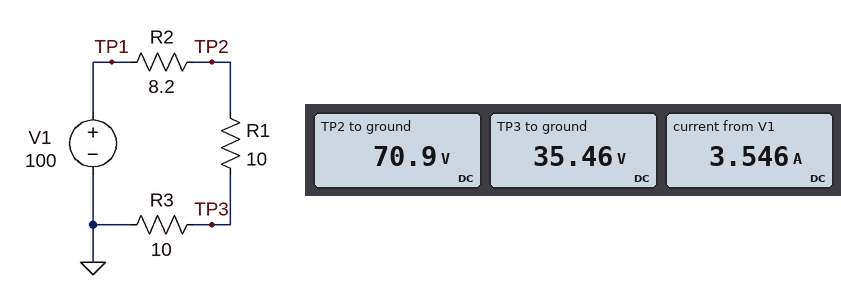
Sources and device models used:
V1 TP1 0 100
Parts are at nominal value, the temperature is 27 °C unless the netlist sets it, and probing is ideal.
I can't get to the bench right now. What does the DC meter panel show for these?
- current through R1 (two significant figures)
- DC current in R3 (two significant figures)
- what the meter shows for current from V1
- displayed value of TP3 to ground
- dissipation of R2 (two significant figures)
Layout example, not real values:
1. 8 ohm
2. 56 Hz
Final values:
1. 3.5 A
2. 3.5 A
3. 3.546 A
4. 35.46 V
5. 100 W
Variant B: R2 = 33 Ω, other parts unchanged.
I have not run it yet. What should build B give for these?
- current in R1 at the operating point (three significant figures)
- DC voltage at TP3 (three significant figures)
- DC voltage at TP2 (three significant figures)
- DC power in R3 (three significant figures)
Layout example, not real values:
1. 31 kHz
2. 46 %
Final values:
1. 1.89 A
2. 18.9 V
3. 37.7 V
4. 35.6 W
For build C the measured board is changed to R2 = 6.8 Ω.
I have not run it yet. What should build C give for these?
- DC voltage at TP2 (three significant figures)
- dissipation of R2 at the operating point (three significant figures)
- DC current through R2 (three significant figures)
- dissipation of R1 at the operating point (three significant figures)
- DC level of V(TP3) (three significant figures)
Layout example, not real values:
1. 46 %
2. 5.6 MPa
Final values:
1. 74.6 V
2. 94.7 W
3. 3.73 A
4. 139 W
5. 37.3 V
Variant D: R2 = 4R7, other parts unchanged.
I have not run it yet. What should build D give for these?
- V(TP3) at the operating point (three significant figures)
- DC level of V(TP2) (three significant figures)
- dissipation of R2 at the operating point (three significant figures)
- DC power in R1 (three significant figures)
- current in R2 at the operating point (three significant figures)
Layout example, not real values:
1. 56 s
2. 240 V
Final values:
1. 40.5 V
2. 81.0 V
3. 77.0 W
4. 164 W
5. 4.05 A
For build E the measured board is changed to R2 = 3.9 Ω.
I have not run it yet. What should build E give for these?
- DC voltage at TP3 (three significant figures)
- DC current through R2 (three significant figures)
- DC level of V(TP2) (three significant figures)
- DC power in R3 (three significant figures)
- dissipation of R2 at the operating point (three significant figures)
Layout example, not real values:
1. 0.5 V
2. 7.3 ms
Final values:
1. 41.8 V
2. 4.18 A
3. 83.7 V
4. 175 W
5. 68.3 W
